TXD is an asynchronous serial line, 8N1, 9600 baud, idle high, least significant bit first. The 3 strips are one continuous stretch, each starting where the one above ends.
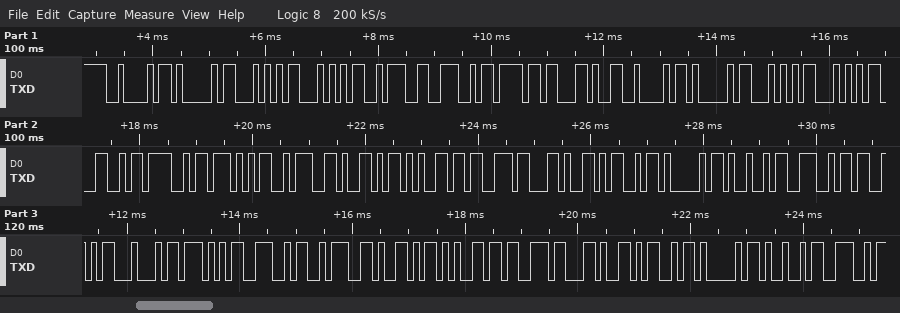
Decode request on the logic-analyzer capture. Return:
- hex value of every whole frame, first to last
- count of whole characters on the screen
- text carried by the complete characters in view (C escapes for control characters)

0x42 0x41 0x54 0x54 0x3A 0x4E 0x6F 0x2C 0x42 0x41 0x54 0x54 0x4C 0x4F 0x57 0x3A 0x59 0x65 0x73 0x2C 0x4D 0x41 0x49 0x4E 0x53 0x44 0x57 0x4E 0x3A 0x59 0x65 0x73 0x2C 0x4D 0x41 0x49 0x4E
37
"BATT:No,BATTLOW:Yes,MAINSDWN:Yes,MAIN"
